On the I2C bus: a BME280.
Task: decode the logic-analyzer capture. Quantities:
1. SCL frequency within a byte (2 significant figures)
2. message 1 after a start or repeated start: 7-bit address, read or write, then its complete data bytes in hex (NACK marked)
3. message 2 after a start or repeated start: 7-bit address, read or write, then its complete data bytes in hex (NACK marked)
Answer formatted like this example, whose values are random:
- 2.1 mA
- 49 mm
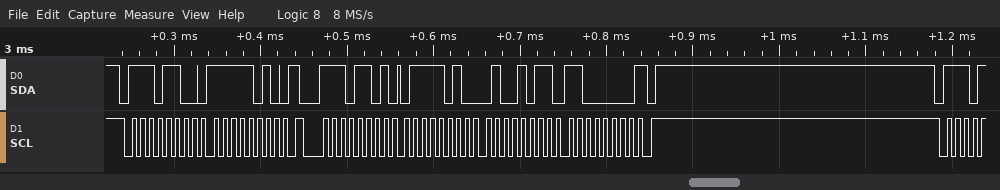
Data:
- 100 kHz
- 0x76 write: FA
- 0x76 read: 7A 4B C0 NACK
